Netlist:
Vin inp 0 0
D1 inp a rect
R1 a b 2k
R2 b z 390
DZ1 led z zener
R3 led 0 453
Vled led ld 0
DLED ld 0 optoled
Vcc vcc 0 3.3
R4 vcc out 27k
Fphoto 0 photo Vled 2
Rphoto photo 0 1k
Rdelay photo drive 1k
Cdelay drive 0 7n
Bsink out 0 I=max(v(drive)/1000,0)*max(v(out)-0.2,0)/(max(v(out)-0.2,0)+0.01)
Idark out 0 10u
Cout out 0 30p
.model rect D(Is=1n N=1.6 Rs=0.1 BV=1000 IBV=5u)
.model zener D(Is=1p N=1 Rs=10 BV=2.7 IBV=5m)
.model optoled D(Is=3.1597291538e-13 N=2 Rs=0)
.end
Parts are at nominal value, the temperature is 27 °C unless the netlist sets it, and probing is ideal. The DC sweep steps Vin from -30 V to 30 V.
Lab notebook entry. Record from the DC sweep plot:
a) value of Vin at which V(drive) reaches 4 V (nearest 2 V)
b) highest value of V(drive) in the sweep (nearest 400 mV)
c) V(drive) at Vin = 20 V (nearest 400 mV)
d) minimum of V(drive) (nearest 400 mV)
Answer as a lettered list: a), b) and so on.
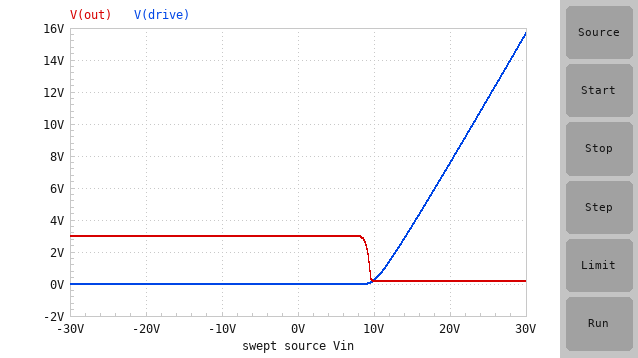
a) 16 V
b) 15.6 V
c) 7.6 V
d) 0 V
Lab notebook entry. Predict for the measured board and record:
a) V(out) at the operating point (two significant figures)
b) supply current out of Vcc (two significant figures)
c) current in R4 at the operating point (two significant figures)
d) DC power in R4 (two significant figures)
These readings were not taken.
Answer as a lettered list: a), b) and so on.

a) 3.0 V
b) 10 µA
c) 10 µA
d) 2.7 µW
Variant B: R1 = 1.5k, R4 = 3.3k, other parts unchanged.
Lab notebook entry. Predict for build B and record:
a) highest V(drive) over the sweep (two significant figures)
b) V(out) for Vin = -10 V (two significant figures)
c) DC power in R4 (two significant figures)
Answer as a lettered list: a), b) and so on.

a) 21 V
b) 3.3 V
c) 330 nW
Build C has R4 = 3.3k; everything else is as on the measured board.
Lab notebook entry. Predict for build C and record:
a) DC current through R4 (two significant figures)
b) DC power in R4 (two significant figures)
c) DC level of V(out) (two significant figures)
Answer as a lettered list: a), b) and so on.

a) 10 µA
b) 330 nW
c) 3.3 V
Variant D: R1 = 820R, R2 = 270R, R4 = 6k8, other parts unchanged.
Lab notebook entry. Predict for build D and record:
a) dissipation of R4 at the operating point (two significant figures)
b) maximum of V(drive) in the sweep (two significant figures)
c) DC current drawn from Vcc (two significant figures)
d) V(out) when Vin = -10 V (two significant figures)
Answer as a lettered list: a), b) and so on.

a) 680 nW
b) 40 V
c) 10 µA
d) 3.2 V
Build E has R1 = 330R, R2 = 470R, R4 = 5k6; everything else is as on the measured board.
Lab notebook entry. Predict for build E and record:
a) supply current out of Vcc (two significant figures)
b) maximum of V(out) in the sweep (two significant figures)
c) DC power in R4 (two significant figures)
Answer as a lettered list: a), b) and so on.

a) 10 µA
b) 3.2 V
c) 560 nW
